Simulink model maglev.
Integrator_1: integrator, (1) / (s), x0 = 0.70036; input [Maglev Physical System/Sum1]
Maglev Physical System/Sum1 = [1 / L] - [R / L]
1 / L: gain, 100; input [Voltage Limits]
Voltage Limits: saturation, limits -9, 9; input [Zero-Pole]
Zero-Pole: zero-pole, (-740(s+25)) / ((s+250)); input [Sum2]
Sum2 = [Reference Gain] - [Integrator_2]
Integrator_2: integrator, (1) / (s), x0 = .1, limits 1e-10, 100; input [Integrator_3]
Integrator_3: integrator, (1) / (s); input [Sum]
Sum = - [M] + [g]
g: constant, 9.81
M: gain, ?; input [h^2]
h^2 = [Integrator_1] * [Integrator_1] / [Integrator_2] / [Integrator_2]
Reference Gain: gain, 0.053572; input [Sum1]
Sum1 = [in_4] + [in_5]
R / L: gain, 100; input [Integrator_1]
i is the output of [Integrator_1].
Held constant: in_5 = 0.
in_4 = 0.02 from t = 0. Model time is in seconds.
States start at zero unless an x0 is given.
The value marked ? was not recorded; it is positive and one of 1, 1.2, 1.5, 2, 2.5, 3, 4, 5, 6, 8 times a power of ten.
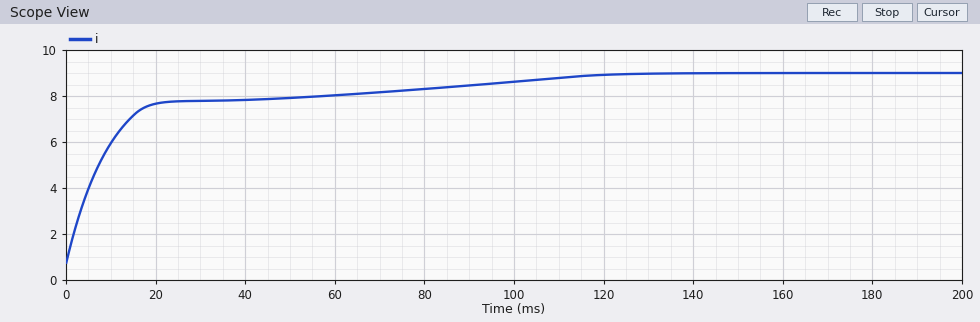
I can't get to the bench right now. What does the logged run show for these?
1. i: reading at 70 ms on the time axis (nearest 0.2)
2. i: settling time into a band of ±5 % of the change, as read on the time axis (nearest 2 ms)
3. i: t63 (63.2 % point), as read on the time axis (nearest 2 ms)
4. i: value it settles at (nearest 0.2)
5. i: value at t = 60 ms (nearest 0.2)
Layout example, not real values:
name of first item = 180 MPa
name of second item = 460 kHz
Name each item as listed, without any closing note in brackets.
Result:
i: reading at 70 ms on the time axis = 8.2
i: settling time into a band of ±5 % of the change, as read on the time axis = 98 ms
i: t63 (63.2 % point), as read on the time axis = 10 ms
i: value it settles at = 9.0
i: value at t = 60 ms = 8.0
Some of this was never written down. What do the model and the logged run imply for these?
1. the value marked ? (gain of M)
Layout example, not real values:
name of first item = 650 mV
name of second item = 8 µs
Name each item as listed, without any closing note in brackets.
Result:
the value marked ? = 0.0015
